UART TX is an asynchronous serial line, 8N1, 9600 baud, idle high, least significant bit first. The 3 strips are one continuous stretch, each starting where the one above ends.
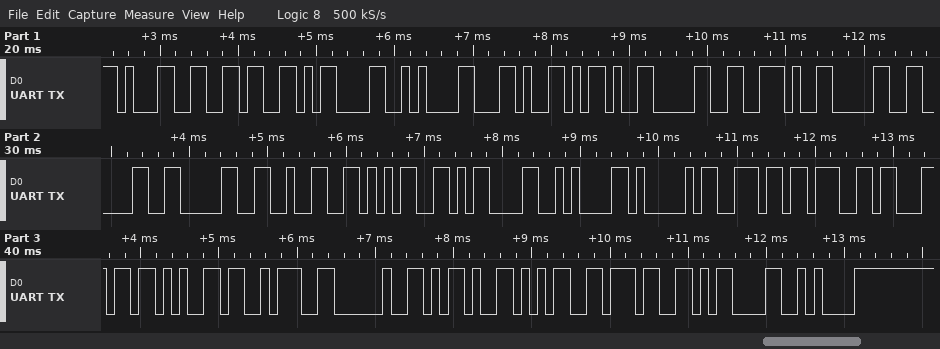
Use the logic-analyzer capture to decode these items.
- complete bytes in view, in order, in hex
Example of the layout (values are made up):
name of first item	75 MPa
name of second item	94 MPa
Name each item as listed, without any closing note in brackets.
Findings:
complete bytes in view, in order, in hex	31 36 0D 0A 2C 2D 30 2E 30 30 30 32 35 0D 0A 41 6E 67 6C 65 3A 20 2D 35 37 0D 0A
